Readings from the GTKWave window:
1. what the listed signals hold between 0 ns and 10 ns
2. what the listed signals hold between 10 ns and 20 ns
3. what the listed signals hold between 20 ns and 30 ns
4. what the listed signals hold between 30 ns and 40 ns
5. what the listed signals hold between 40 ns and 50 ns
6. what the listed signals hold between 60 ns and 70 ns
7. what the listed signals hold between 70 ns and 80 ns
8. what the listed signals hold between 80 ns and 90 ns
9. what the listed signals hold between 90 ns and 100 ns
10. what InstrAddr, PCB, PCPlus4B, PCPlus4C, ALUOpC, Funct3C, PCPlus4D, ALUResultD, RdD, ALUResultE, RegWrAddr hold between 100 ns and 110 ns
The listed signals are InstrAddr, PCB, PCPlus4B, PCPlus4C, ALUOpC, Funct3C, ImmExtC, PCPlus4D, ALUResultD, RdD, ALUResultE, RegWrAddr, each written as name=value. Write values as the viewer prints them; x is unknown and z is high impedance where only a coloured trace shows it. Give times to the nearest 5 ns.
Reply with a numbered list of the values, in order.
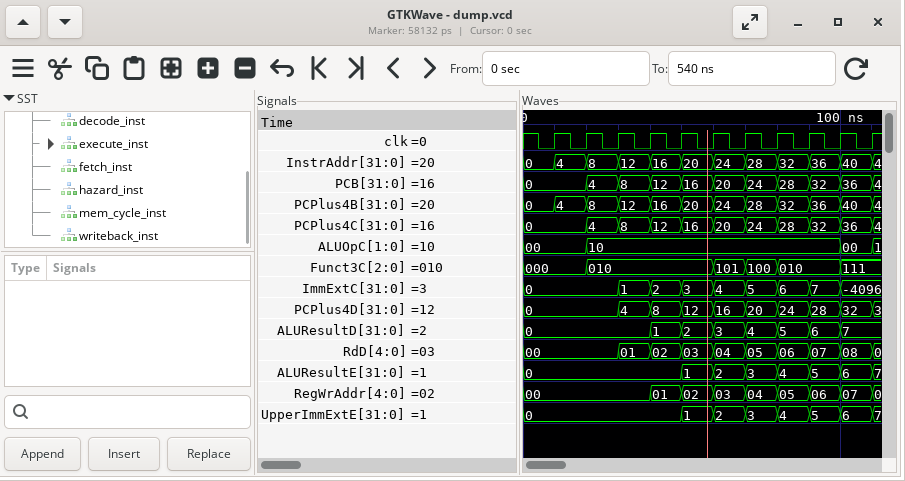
1. InstrAddr=0, PCB=0, PCPlus4B=0, PCPlus4C=0, ALUOpC=00, Funct3C=000, ImmExtC=0, PCPlus4D=0, ALUResultD=0, RdD=00, ALUResultE=0, RegWrAddr=00
2. InstrAddr=4, PCB=0, PCPlus4B=4, PCPlus4C=0, ALUOpC=00, Funct3C=000, ImmExtC=0, PCPlus4D=0, ALUResultD=0, RdD=00, ALUResultE=0, RegWrAddr=00
3. InstrAddr=8, PCB=4, PCPlus4B=8, PCPlus4C=4, ALUOpC=10, Funct3C=010, ImmExtC=0, PCPlus4D=0, ALUResultD=0, RdD=00, ALUResultE=0, RegWrAddr=00
4. InstrAddr=12, PCB=8, PCPlus4B=12, PCPlus4C=8, ALUOpC=10, Funct3C=010, ImmExtC=1, PCPlus4D=4, ALUResultD=0, RdD=01, ALUResultE=0, RegWrAddr=00
5. InstrAddr=16, PCB=12, PCPlus4B=16, PCPlus4C=12, ALUOpC=10, Funct3C=010, ImmExtC=2, PCPlus4D=8, ALUResultD=1, RdD=02, ALUResultE=0, RegWrAddr=01
6. InstrAddr=24, PCB=20, PCPlus4B=24, PCPlus4C=20, ALUOpC=10, Funct3C=101, ImmExtC=4, PCPlus4D=16, ALUResultD=3, RdD=04, ALUResultE=2, RegWrAddr=03
7. InstrAddr=28, PCB=24, PCPlus4B=28, PCPlus4C=24, ALUOpC=10, Funct3C=100, ImmExtC=5, PCPlus4D=20, ALUResultD=4, RdD=05, ALUResultE=3, RegWrAddr=04
8. InstrAddr=32, PCB=28, PCPlus4B=32, PCPlus4C=28, ALUOpC=10, Funct3C=010, ImmExtC=6, PCPlus4D=24, ALUResultD=5, RdD=06, ALUResultE=4, RegWrAddr=05
9. InstrAddr=36, PCB=32, PCPlus4B=36, PCPlus4C=32, ALUOpC=10, Funct3C=010, ImmExtC=7, PCPlus4D=28, ALUResultD=6, RdD=07, ALUResultE=5, RegWrAddr=06
10. InstrAddr=40, PCB=36, PCPlus4B=40, PCPlus4C=36, ALUOpC=00, Funct3C=111, PCPlus4D=32, ALUResultD=7, RdD=08, ALUResultE=6, RegWrAddr=07
